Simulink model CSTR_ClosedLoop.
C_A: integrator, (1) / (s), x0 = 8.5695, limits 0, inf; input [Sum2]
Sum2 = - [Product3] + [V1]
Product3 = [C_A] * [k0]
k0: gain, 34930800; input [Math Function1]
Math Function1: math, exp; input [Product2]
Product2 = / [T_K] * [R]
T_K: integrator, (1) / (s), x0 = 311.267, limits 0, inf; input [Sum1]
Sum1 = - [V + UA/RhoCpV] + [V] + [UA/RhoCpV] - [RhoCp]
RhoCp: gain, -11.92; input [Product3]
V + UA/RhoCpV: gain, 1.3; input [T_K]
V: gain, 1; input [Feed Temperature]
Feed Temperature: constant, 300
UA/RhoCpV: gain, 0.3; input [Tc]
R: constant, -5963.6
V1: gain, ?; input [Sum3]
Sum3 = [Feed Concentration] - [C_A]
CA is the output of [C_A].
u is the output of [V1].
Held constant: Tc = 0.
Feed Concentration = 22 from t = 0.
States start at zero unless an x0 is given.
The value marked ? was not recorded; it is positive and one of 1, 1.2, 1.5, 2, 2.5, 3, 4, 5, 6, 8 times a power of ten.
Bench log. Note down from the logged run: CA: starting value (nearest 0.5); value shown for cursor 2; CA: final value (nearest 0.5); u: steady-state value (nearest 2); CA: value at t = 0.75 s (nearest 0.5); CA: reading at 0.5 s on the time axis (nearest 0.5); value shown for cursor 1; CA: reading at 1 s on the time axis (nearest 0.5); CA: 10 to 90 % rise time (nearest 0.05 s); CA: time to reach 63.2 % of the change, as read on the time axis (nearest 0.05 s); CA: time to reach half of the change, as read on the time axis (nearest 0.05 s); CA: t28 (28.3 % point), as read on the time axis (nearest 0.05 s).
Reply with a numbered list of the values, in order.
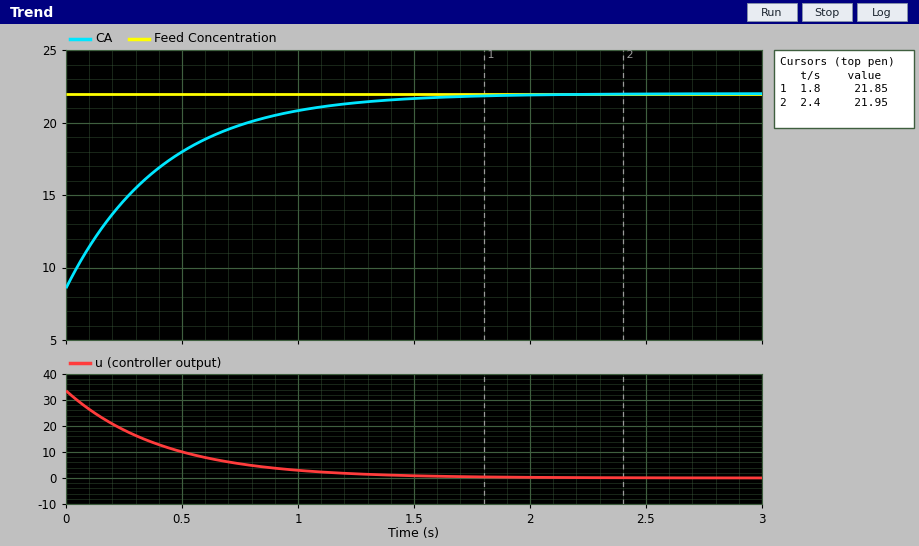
1. 8.5
2. 21.95
3. 22.0
4. 0
5. 20.0
6. 18.0
7. 21.85
8. 21.0
9. 0.90 s
10. 0.40 s
11. 0.30 s
12. 0.15 s
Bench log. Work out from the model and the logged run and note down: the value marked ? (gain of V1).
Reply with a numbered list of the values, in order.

1. 2.5
